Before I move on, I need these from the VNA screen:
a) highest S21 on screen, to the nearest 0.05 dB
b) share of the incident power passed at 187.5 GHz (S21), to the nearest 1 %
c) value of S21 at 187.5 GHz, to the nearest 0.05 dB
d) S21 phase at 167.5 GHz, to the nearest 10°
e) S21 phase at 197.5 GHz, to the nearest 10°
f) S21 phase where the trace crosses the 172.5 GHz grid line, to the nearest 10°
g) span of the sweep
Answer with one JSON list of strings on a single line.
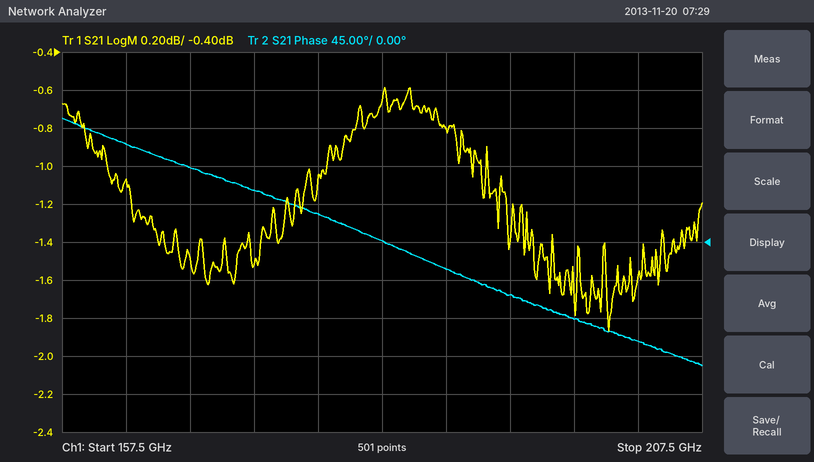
["-0.60 dB", "83 %", "-0.80 dB", "90°", "-90°", "60°", "50 GHz"]
